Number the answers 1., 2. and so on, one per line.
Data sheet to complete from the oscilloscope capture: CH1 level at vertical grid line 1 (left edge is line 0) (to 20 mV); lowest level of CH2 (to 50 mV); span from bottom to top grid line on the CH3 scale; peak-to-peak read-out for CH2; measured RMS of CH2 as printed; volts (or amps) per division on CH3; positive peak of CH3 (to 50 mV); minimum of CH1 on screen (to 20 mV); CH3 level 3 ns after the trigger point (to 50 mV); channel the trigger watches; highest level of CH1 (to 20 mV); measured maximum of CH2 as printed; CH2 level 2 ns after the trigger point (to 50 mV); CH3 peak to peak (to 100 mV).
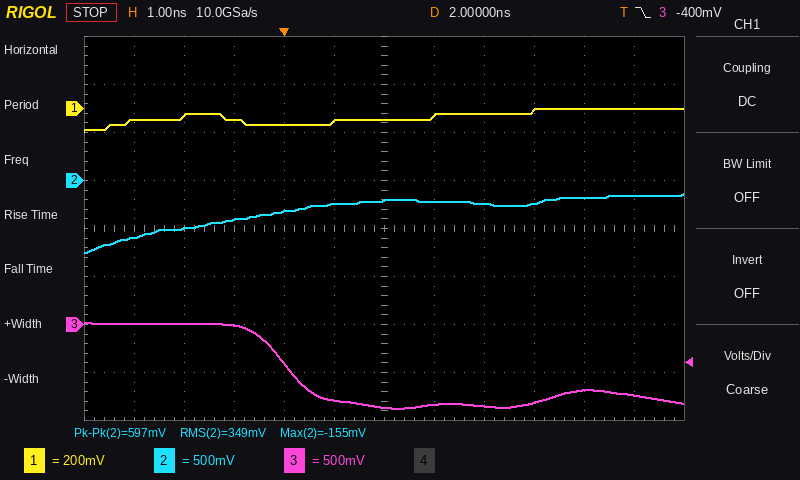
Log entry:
1. -40 mV
2. -750 mV
3. 4 V
4. 597 mV
5. 349 mV
6. 500 mV
7. 0 mV
8. -100 mV
9. -850 mV
10. CH3
11. 0 mV
12. -155 mV
13. -200 mV
14. 900 mV
